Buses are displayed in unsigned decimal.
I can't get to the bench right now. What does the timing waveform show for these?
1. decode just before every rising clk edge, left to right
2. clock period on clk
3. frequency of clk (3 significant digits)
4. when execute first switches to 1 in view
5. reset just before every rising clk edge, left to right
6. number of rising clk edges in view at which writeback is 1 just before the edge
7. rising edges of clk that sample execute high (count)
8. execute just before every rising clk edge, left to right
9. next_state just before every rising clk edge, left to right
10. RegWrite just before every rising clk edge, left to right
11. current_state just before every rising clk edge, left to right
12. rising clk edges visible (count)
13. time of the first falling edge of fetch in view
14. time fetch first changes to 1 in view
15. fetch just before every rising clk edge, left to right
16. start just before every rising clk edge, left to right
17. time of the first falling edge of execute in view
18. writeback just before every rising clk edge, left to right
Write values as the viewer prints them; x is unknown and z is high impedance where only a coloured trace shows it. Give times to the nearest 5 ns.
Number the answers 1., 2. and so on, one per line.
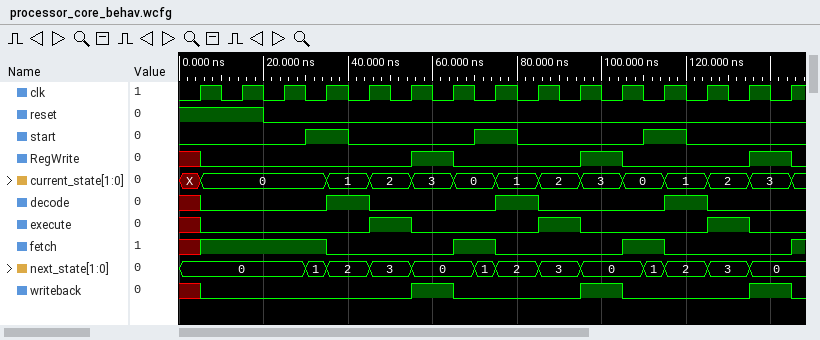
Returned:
1. x 0 0 0 1 0 0 0 1 0 0 0 1 0 0
2. 10 ns
3. 100 MHz
4. 45 ns
5. 1 1 0 0 0 0 0 0 0 0 0 0 0 0 0
6. 3
7. 3
8. x 0 0 0 0 1 0 0 0 1 0 0 0 1 0
9. 0, 0, 0, 1, 2, 3, 0, 1, 2, 3, 0, 1, 2, 3, 0
10. x 0 0 0 0 0 1 0 0 0 1 0 0 0 1
11. X, 0, 0, 0, 1, 2, 3, 0, 1, 2, 3, 0, 1, 2, 3
12. 15
13. 35 ns
14. 5 ns
15. x 1 1 1 0 0 0 1 0 0 0 1 0 0 0
16. 0 0 0 1 0 0 0 1 0 0 0 1 0 0 0
17. 55 ns
18. x 0 0 0 0 0 1 0 0 0 1 0 0 0 1
